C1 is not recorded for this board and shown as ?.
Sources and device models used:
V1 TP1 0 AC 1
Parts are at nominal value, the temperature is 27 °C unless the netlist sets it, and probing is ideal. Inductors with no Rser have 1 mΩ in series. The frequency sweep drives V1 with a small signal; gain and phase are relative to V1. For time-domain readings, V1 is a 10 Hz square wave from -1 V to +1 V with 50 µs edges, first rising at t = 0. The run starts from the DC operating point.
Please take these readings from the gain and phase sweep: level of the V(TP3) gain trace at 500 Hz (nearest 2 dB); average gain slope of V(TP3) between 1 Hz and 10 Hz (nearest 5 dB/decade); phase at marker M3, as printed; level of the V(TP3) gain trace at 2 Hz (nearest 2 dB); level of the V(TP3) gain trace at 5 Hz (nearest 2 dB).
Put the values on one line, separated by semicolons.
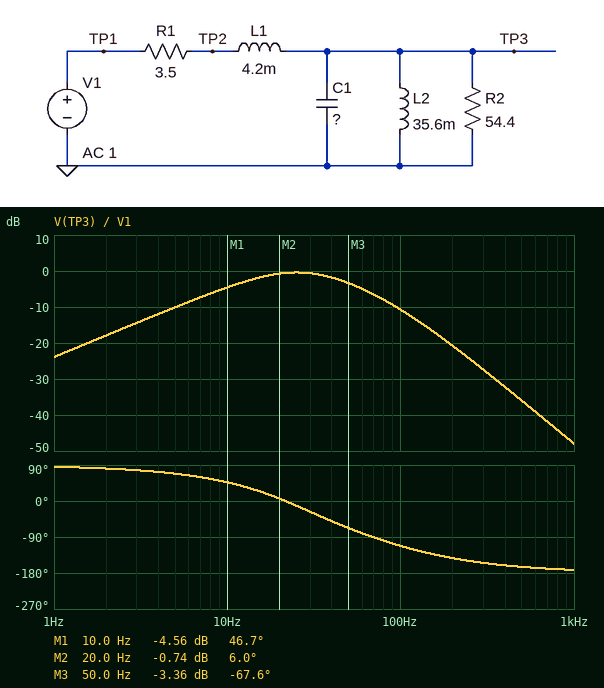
-36 dB; 20 dB/decade; -67.6 deg; -18 dB; -10 dB
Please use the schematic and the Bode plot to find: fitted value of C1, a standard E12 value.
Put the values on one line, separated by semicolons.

1.5 mF
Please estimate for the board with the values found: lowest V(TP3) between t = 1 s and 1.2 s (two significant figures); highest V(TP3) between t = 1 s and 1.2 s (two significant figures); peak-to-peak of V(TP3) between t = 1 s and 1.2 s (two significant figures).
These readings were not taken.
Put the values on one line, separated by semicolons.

-1.3 V; 1.3 V; 2.6 V
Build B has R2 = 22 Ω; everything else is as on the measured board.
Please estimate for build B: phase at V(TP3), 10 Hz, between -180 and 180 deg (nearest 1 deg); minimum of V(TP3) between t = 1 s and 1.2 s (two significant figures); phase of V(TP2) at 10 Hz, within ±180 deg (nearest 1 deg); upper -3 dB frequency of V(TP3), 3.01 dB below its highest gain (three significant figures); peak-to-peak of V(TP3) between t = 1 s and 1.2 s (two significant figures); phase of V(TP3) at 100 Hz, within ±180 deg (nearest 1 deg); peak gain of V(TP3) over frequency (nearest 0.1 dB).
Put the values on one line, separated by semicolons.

44 deg; -1.2 V; 45 deg; 52.8 Hz; 2.5 V; -110 deg; -1.2 dB
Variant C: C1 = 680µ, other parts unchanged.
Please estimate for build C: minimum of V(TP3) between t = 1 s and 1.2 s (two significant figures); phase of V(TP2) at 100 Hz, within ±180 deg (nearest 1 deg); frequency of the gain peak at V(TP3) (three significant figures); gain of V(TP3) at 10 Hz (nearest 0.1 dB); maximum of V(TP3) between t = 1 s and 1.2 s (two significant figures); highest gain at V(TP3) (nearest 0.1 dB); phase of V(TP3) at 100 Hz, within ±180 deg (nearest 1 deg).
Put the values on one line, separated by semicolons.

-1.6 V; 13 deg; 50.7 Hz; -5.3 dB; 1.6 V; -0.1 dB; -88 deg
